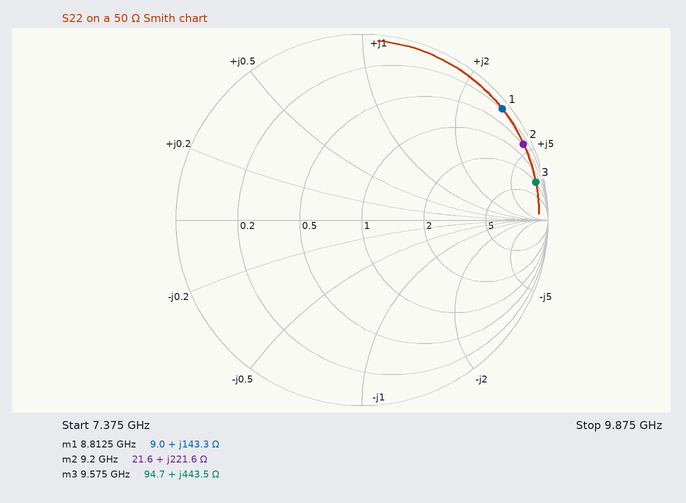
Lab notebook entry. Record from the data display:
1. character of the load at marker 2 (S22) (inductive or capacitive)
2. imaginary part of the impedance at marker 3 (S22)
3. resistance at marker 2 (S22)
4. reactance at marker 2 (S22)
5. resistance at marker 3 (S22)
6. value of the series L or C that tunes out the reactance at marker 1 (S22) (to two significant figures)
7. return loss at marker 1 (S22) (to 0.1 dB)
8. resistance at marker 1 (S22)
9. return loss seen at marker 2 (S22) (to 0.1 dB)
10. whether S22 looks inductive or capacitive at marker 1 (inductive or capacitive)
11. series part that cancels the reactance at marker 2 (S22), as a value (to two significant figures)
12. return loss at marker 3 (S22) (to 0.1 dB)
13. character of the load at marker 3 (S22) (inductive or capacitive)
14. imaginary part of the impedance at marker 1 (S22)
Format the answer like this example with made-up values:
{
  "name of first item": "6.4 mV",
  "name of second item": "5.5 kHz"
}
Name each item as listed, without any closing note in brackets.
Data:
{
  "character of the load at marker 2 (S22)": "inductive",
  "imaginary part of the impedance at marker 3": "+443.5 Ω",
  "resistance at marker 2": "21.6 Ω",
  "reactance at marker 2": "+221.6 Ω",
  "resistance at marker 3": "94.7 Ω",
  "value of the series L or C that tunes out the reactance at marker 1 (S22)": "130 fF",
  "return loss at marker 1 (S22)": "0.3 dB",
  "resistance at marker 1": "9.0 Ω",
  "return loss seen at marker 2 (S22)": "0.4 dB",
  "whether S22 looks inductive or capacitive at marker 1": "inductive",
  "series part that cancels the reactance at marker 2 (S22), as a value": "78 fF",
  "return loss at marker 3 (S22)": "0.4 dB",
  "character of the load at marker 3 (S22)": "inductive",
  "imaginary part of the impedance at marker 1": "+143.3 Ω"
}
